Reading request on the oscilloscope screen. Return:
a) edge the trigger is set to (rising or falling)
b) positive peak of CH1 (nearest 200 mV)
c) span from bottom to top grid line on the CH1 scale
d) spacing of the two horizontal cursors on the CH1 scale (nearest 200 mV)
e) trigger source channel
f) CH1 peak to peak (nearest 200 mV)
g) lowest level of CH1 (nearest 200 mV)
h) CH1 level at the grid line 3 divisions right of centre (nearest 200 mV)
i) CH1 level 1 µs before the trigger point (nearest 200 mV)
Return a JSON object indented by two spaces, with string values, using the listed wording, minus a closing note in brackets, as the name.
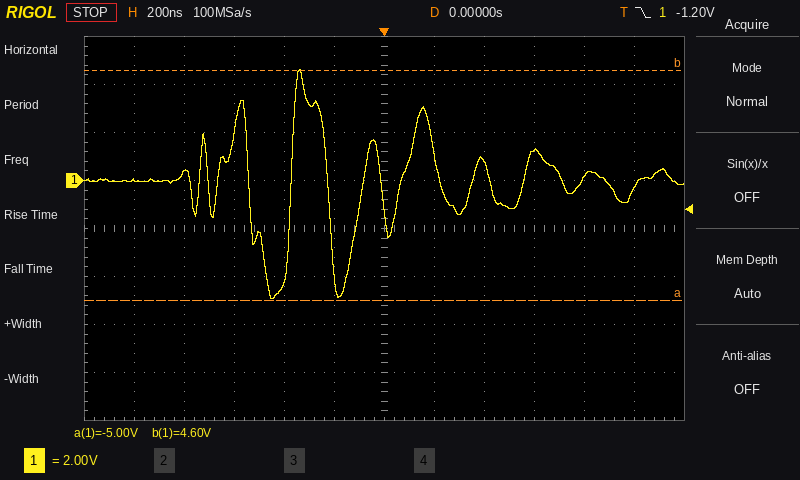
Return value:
{
  "edge the trigger is set to": "falling",
  "positive peak of CH1": "4.6 V",
  "span from bottom to top grid line on the CH1 scale": "16 V",
  "spacing of the two horizontal cursors on the CH1 scale": "9.6 V",
  "trigger source channel": "CH1",
  "CH1 peak to peak": "9.6 V",
  "lowest level of CH1": "-5.0 V",
  "CH1 level at the grid line 3 divisions right of centre": "1.2 V",
  "CH1 level 1 µs before the trigger point": "0.0 V"
}
